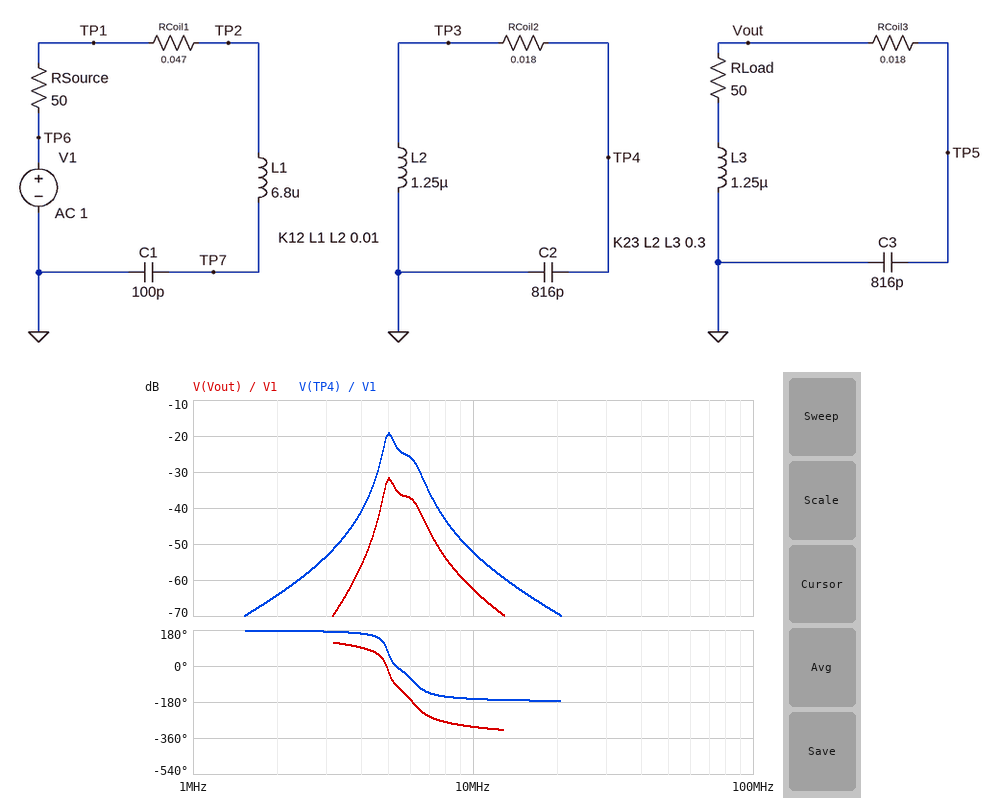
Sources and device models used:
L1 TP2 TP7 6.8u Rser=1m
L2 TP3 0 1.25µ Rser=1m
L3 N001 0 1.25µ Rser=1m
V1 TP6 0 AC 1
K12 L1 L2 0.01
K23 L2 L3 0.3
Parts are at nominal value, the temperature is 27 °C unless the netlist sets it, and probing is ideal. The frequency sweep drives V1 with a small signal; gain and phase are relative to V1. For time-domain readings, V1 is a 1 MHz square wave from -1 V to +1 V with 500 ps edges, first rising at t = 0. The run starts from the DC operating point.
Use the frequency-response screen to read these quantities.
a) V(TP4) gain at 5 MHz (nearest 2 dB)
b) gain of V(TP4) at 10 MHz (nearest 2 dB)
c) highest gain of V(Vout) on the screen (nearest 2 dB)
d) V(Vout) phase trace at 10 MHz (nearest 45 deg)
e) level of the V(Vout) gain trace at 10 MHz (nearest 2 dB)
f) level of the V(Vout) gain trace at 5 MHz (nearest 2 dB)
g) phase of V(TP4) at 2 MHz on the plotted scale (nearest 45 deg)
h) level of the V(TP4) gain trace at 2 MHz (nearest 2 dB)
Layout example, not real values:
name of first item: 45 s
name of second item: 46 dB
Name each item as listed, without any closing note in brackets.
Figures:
V(TP4) gain at 5 MHz: -20 dB
gain of V(TP4) at 10 MHz: -52 dB
highest gain of V(Vout) on the screen: -32 dB
V(Vout) phase trace at 10 MHz: -315 deg
level of the V(Vout) gain trace at 10 MHz: -62 dB
level of the V(Vout) gain trace at 5 MHz: -32 dB
phase of V(TP4) at 2 MHz on the plotted scale: 180 deg
level of the V(TP4) gain trace at 2 MHz: -64 dB
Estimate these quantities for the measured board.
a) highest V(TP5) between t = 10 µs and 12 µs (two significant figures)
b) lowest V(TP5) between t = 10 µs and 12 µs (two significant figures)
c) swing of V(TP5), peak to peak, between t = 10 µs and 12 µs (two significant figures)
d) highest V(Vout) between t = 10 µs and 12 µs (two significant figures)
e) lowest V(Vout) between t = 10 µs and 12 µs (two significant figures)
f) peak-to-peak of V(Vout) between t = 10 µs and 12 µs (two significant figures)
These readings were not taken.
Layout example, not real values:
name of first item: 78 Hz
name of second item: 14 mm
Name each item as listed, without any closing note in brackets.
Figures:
highest V(TP5) between t = 10 µs and 12 µs: 7.3 mV
lowest V(TP5) between t = 10 µs and 12 µs: -7.3 mV
swing of V(TP5), peak to peak, between t = 10 µs and 12 µs: 15 mV
highest V(Vout) between t = 10 µs and 12 µs: 7.3 mV
lowest V(Vout) between t = 10 µs and 12 µs: -7.3 mV
peak-to-peak of V(Vout) between t = 10 µs and 12 µs: 15 mV
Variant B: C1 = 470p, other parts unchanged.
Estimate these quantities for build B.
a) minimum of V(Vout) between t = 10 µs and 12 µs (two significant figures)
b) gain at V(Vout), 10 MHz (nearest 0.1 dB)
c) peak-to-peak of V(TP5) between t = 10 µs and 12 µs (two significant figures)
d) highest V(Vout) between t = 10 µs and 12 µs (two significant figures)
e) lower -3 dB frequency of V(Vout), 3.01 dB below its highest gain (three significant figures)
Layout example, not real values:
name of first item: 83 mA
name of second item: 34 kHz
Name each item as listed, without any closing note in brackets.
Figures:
minimum of V(Vout) between t = 10 µs and 12 µs: -5.8 mV
gain at V(Vout), 10 MHz: -65.8 dB
peak-to-peak of V(TP5) between t = 10 µs and 12 µs: 12 mV
highest V(Vout) between t = 10 µs and 12 µs: 5.8 mV
lower -3 dB frequency of V(Vout), 3.01 dB below its highest gain: 4.78 MHz
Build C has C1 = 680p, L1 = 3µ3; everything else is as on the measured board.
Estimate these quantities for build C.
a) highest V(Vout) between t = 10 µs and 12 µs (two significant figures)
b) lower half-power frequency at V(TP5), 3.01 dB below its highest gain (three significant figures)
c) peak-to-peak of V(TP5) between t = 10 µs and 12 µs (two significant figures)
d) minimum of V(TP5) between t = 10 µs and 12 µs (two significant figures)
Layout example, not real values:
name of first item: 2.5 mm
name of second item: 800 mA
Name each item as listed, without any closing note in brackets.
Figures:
highest V(Vout) between t = 10 µs and 12 µs: 7.7 mV
lower half-power frequency at V(TP5), 3.01 dB below its highest gain: 4.78 MHz
peak-to-peak of V(TP5) between t = 10 µs and 12 µs: 15 mV
minimum of V(TP5) between t = 10 µs and 12 µs: -7.7 mV
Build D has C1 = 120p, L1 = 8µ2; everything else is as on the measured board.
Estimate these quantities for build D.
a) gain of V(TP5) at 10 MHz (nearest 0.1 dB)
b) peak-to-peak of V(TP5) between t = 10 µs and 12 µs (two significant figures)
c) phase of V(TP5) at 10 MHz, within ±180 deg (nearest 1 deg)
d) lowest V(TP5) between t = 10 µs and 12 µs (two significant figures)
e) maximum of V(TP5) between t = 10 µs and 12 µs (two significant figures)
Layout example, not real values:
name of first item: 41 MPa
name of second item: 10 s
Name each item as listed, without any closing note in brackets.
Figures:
gain of V(TP5) at 10 MHz: -64.8 dB
peak-to-peak of V(TP5) between t = 10 µs and 12 µs: 34 mV
phase of V(TP5) at 10 MHz, within ±180 deg: 53 deg
lowest V(TP5) between t = 10 µs and 12 µs: -17 mV
maximum of V(TP5) between t = 10 µs and 12 µs: 17 mV
